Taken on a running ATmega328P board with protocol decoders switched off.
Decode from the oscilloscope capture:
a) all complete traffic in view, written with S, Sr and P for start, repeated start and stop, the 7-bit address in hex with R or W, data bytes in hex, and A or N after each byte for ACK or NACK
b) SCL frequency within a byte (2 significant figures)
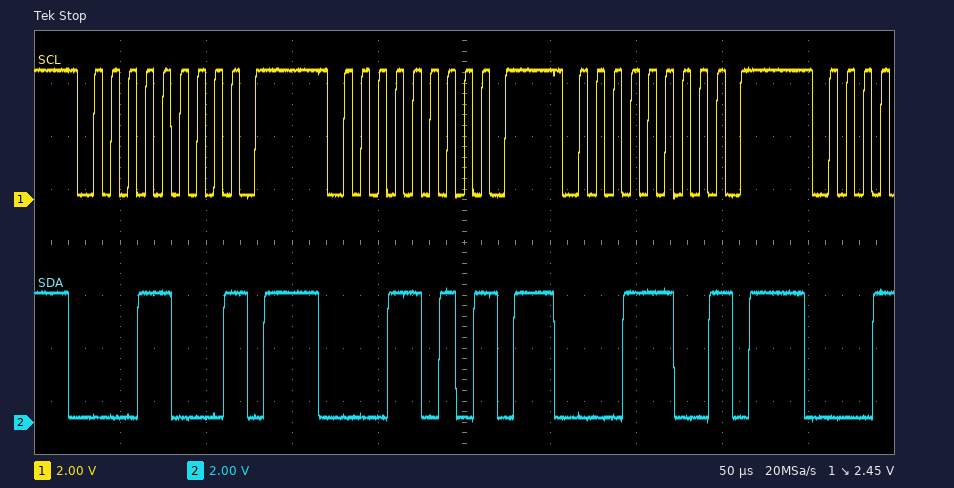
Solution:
S 0CW N P S 0DW N P S 0EW N P
100 kHz
